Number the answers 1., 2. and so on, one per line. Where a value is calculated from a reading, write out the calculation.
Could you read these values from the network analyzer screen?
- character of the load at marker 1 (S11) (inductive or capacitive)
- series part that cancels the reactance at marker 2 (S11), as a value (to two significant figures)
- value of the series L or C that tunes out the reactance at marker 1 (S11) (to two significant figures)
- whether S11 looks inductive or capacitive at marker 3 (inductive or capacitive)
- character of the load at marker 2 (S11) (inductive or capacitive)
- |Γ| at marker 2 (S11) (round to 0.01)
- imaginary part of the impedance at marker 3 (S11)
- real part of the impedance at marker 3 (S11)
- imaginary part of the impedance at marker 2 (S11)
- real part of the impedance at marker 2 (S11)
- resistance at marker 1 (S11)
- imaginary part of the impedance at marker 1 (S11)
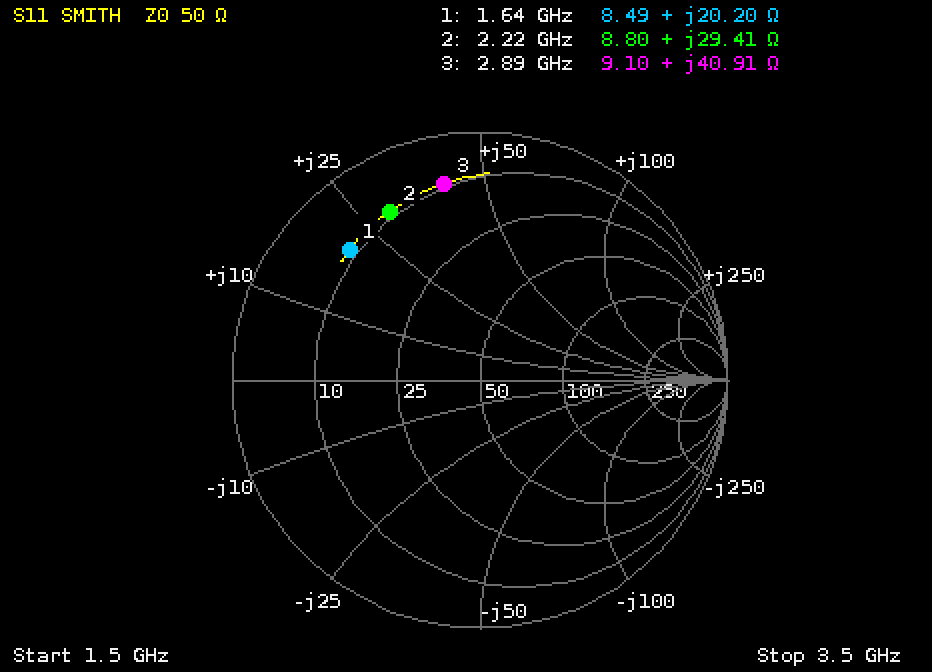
1. inductive
2. C = 1/(2π × 2.22 GHz × 29.41 Ω) ≈ 2.4 pF
3. C = 1/(2π × 1.64 GHz × 20.2 Ω) ≈ 4.8 pF
4. inductive
5. inductive
6. 0.77
7. +40.91 Ω
8. 9.10 Ω
9. +29.41 Ω
10. 8.80 Ω
11. 8.49 Ω
12. +20.20 Ω
